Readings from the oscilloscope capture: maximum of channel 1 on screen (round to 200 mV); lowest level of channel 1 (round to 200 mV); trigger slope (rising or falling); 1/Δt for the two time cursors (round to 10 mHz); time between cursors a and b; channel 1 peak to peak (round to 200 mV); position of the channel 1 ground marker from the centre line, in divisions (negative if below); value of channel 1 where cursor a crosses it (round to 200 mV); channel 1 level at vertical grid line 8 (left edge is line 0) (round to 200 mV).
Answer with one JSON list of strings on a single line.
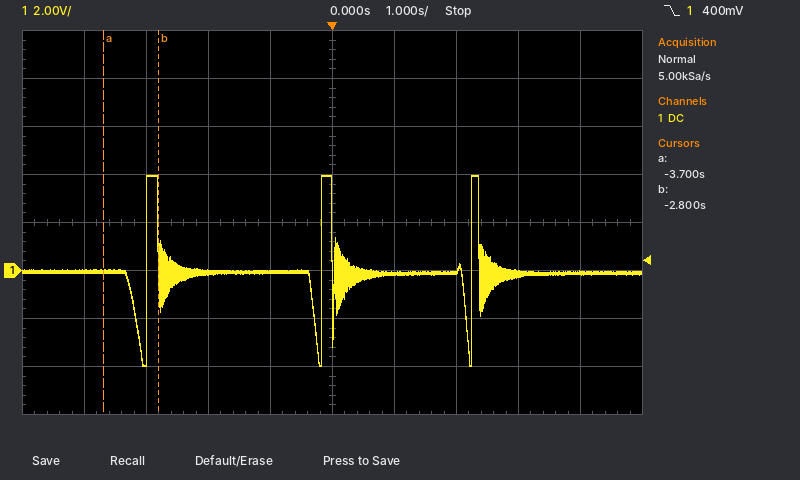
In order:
["4.0 V", "-4.0 V", "falling", "1.11 Hz", "900 ms", "8.0 V", "-1.0 div", "0.0 V", "-200 mV"]
